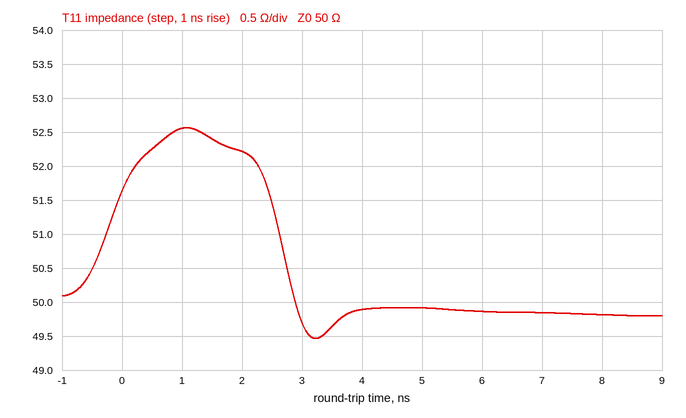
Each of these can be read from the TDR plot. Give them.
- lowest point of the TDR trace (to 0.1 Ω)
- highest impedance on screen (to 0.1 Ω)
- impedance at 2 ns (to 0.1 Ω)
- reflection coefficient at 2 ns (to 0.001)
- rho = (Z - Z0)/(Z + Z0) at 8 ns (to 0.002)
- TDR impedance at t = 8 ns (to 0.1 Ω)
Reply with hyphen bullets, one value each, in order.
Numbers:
- 49.5 Ω
- 52.6 Ω
- 52.2 Ω
- +0.022
- -0.002
- 49.8 Ω
